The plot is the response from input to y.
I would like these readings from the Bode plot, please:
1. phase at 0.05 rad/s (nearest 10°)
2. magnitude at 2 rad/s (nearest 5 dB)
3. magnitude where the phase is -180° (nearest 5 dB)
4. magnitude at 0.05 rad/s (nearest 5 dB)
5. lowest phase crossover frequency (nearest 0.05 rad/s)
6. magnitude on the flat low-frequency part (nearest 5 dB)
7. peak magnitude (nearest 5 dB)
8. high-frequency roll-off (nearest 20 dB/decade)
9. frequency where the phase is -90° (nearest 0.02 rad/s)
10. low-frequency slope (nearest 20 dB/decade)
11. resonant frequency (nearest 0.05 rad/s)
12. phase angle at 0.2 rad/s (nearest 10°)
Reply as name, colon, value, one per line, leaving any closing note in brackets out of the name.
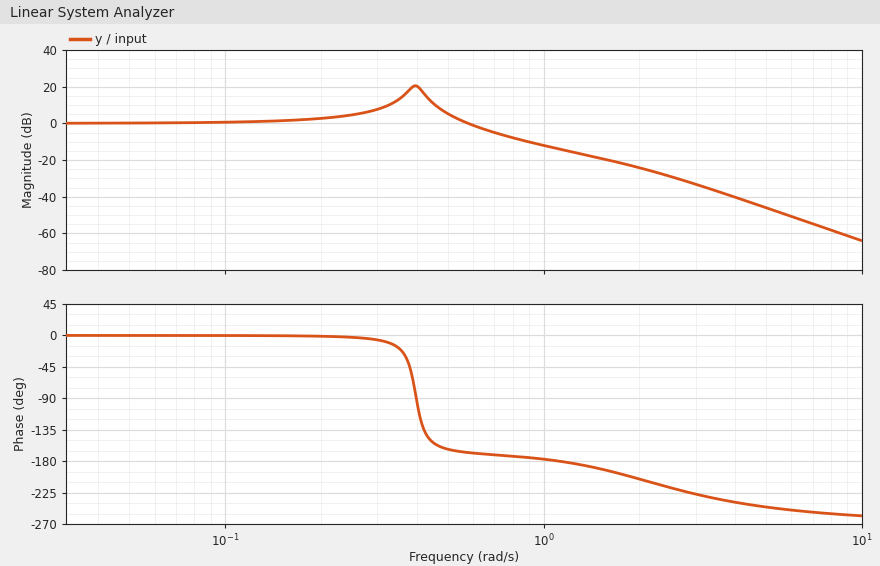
phase at 0.05 rad/s: 0°
magnitude at 2 rad/s: -25 dB
magnitude where the phase is -180°: -15 dB
magnitude at 0.05 rad/s: 0 dB
lowest phase crossover frequency: 1.10 rad/s
magnitude on the flat low-frequency part: 0 dB
peak magnitude: 20 dB
high-frequency roll-off: -60 dB/decade
frequency where the phase is -90°: 0.40 rad/s
low-frequency slope: 0 dB/decade
resonant frequency: 0.40 rad/s
phase angle at 0.2 rad/s: 0°
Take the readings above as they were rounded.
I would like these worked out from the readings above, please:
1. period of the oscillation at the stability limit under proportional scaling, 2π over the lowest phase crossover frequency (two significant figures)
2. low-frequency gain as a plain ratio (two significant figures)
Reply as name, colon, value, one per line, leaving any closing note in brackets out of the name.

period of the oscillation at the stability limit under proportional scaling, 2π over the lowest phase crossover frequency: 5.7 s
low-frequency gain as a plain ratio: 1.0
